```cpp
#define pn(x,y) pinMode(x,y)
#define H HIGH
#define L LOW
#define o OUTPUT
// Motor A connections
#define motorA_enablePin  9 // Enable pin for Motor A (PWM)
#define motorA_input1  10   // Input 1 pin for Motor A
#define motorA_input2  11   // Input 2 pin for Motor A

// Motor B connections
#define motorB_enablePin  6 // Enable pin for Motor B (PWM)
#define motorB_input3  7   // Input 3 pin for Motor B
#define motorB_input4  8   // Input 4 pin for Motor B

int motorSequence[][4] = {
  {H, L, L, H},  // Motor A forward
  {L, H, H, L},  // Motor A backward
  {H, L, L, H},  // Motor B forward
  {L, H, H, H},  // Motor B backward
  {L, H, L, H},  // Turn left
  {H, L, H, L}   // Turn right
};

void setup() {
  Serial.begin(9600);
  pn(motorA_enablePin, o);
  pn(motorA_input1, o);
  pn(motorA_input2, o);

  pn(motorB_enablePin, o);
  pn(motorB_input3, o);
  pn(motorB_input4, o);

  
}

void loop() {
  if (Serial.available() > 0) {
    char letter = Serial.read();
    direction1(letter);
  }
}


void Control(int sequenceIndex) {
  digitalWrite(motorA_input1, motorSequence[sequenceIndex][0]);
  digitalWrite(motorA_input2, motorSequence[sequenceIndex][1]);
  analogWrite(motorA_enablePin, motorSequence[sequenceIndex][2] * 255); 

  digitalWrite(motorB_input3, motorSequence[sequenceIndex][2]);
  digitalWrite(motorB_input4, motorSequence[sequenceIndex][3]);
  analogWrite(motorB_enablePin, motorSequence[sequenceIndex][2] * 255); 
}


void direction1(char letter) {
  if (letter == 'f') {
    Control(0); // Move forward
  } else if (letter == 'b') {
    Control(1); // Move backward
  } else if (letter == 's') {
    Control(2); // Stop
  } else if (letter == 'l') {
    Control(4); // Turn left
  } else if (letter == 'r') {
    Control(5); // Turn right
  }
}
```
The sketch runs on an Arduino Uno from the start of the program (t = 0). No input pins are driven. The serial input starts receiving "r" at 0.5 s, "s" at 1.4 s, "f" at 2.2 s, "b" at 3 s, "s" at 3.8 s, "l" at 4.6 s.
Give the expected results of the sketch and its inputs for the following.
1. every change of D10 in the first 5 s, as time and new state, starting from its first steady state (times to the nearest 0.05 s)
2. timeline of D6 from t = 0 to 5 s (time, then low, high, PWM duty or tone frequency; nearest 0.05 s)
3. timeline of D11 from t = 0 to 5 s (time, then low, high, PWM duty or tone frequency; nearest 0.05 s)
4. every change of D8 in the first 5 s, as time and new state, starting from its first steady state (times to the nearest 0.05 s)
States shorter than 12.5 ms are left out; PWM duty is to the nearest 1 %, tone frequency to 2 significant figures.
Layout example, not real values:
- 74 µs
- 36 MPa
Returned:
- 0 s low; 0.5 s high; 3 s low; 3.8 s high; 4.6 s low
- 0 s low; 0.5 s high; 1.4 s low; 3 s high; 3.8 s low
- 0 s low; 3 s high; 3.8 s low; 4.6 s high
- 0 s low; 1.4 s high; 3 s low; 3.8 s high
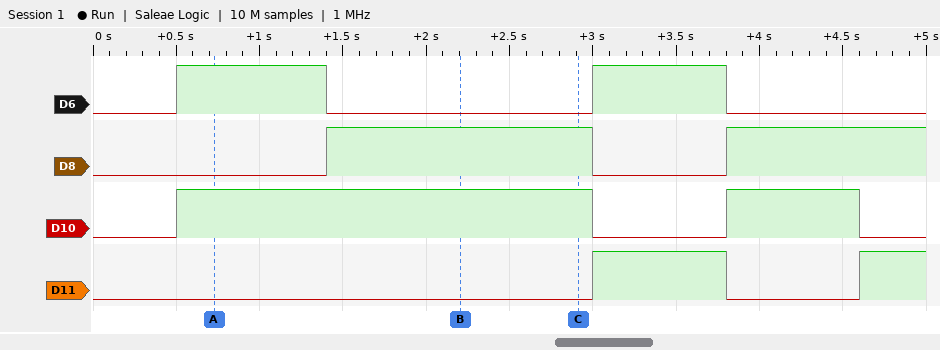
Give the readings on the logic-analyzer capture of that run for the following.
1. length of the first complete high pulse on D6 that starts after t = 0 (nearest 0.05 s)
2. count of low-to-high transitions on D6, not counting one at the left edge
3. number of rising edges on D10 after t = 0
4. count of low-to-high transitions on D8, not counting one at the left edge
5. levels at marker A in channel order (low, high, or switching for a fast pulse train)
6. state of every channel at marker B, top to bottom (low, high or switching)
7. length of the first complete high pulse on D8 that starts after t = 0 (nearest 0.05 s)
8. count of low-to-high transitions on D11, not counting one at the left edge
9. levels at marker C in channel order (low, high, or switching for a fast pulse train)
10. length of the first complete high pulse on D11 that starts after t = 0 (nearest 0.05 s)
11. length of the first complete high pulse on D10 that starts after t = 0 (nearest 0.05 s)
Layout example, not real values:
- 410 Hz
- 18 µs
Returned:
- 0.90 s
- 2
- 2
- 2
- D6 high, D8 low, D10 high, D11 low
- D6 low, D8 high, D10 high, D11 low
- 1.60 s
- 2
- D6 low, D8 high, D10 high, D11 low
- 0.80 s
- 2.50 s
